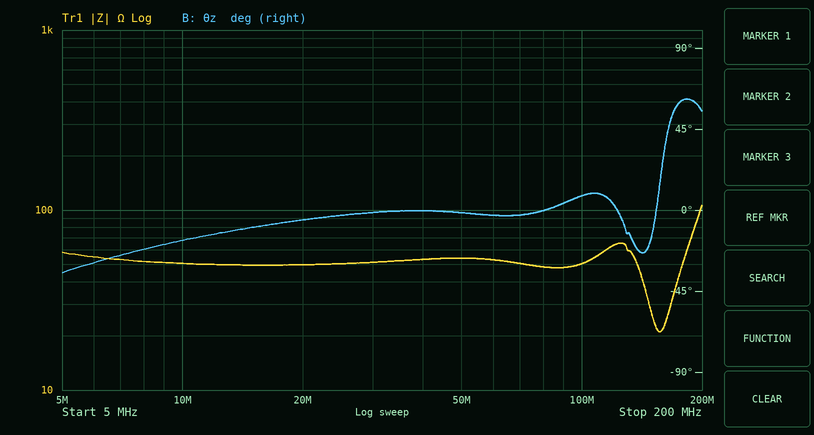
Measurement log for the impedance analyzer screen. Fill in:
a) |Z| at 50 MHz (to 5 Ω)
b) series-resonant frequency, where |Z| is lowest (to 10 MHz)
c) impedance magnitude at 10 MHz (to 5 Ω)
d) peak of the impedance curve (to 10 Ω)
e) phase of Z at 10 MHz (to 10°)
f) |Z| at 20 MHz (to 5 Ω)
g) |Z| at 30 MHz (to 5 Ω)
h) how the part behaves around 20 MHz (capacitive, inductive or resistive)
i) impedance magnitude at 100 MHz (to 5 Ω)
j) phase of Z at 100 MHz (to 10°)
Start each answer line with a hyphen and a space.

- 55 Ω
- 160 MHz
- 50 Ω
- 110 Ω
- -20°
- 50 Ω
- 50 Ω
- resistive
- 50 Ω
- 10°
